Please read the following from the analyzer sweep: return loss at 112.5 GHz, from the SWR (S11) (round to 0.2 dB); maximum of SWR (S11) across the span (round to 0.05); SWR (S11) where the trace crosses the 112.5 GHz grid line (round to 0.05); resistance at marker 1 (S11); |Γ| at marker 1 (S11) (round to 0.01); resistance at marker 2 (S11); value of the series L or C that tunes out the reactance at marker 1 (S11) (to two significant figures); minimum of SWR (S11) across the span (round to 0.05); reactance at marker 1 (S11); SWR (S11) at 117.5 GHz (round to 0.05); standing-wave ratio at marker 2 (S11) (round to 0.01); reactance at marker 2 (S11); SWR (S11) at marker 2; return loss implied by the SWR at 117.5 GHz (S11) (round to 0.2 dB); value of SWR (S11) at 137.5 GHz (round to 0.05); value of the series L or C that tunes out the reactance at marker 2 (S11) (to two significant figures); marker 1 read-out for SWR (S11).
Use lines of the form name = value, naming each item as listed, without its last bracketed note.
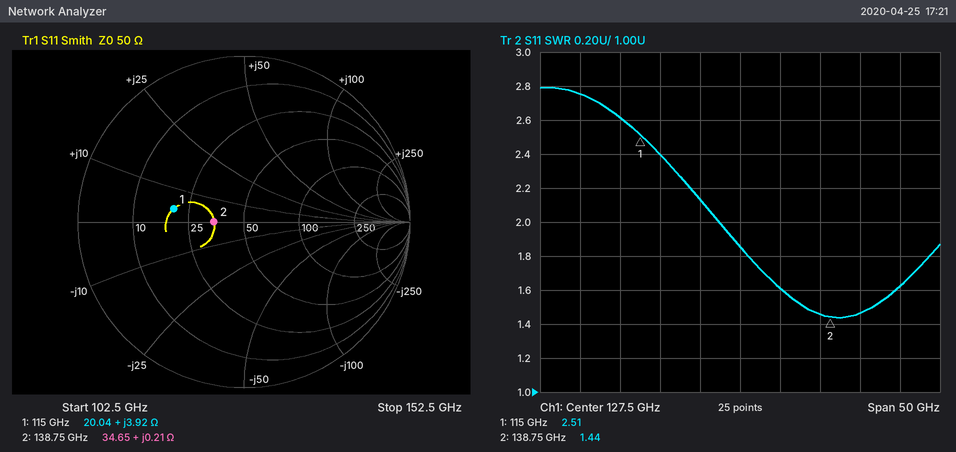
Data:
return loss at 112.5 GHz, from the SWR (S11) = 7.0 dB
maximum of SWR (S11) across the span = 2.80
SWR (S11) where the trace crosses the 112.5 GHz grid line = 2.60
resistance at marker 1 = 20.04 Ω
|Γ| at marker 1 (S11) = 0.43
resistance at marker 2 = 34.65 Ω
value of the series L or C that tunes out the reactance at marker 1 (S11) = 350 fF
minimum of SWR (S11) across the span = 1.45
reactance at marker 1 = +3.92 Ω
SWR (S11) at 117.5 GHz = 2.40
standing-wave ratio at marker 2 (S11) = 1.44
reactance at marker 2 = +0.21 Ω
SWR (S11) at marker 2 = 1.44
return loss implied by the SWR at 117.5 GHz (S11) = 7.8 dB
value of SWR (S11) at 137.5 GHz = 1.45
value of the series L or C that tunes out the reactance at marker 2 (S11) = 5.5 pF
marker 1 read-out for SWR = 2.51
